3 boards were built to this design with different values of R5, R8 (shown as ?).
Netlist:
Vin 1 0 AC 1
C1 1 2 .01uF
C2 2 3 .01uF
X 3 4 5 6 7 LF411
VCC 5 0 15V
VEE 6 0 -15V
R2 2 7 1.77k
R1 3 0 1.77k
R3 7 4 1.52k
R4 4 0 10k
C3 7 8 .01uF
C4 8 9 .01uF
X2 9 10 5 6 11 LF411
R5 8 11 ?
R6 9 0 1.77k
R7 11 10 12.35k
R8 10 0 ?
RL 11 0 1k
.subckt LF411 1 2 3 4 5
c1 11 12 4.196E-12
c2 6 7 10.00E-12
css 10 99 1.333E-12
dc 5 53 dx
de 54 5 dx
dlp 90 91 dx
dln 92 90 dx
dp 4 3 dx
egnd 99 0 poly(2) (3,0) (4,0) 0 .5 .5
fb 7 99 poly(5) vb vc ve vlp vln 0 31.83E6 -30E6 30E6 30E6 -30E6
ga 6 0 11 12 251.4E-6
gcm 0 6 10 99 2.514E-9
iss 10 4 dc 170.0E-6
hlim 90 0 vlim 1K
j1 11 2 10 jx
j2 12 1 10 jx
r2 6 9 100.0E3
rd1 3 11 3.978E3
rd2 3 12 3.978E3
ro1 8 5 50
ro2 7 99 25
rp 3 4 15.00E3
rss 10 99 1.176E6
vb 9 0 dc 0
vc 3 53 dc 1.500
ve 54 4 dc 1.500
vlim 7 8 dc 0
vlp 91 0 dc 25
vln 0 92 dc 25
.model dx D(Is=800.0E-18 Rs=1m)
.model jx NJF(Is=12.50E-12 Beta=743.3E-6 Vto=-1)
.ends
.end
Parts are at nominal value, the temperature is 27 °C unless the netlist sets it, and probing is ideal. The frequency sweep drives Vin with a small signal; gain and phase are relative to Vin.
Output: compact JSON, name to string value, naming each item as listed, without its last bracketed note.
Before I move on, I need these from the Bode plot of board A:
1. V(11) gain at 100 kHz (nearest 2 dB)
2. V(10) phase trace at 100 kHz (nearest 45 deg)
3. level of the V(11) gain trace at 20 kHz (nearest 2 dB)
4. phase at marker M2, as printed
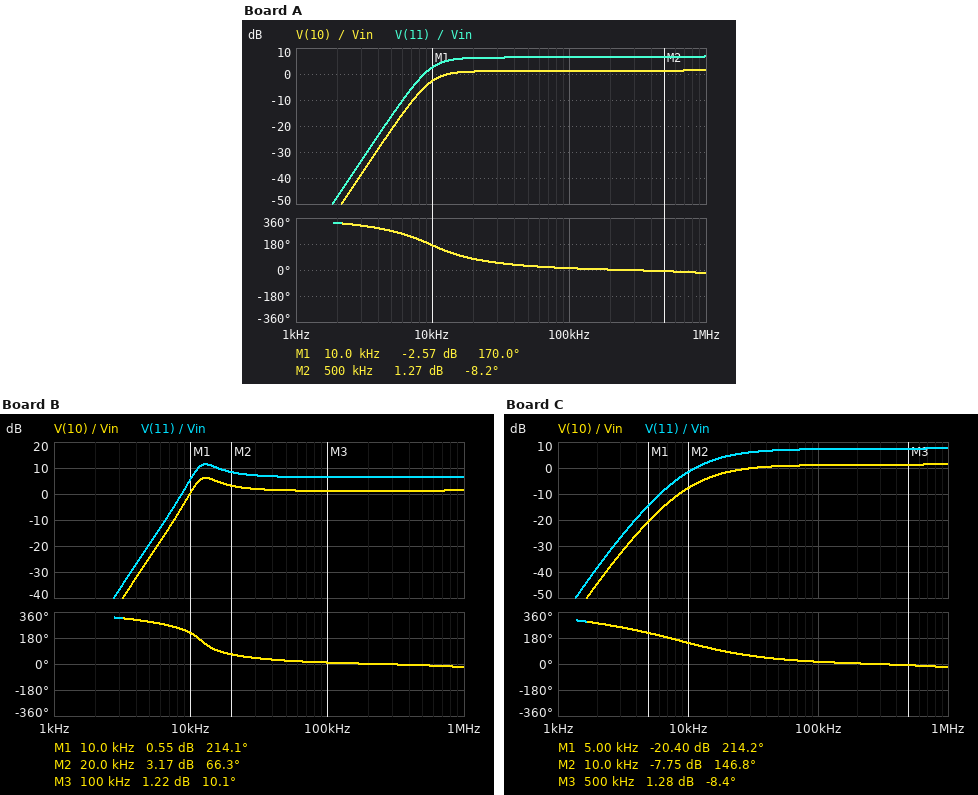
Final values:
{"V(11) gain at 100 kHz": "6 dB", "V(10) phase trace at 100 kHz": "0 deg", "level of the V(11) gain trace at 20 kHz": "6 dB", "phase at marker M2, as printed": "-8.2 deg"}
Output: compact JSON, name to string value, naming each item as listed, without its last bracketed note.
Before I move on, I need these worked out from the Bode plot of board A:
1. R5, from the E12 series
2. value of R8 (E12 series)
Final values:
{"R5, from the E12 series": "1.5 kΩ", "value of R8": "15 kΩ"}
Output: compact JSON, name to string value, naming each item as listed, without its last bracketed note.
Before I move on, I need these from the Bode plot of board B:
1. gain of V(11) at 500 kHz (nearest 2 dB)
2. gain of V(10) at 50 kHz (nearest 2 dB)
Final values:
{"gain of V(11) at 500 kHz": "6 dB", "gain of V(10) at 50 kHz": "2 dB"}
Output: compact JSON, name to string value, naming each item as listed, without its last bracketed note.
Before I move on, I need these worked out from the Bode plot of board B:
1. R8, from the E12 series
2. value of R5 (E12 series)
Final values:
{"R8, from the E12 series": "15 kΩ", "value of R5": "1 kΩ"}
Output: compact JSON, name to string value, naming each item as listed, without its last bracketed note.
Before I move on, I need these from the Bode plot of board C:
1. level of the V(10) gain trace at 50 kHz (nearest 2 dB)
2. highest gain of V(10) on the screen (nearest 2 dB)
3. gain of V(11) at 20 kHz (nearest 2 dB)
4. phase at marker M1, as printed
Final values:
{"level of the V(10) gain trace at 50 kHz": "0 dB", "highest gain of V(10) on the screen": "2 dB", "gain of V(11) at 20 kHz": "4 dB", "phase at marker M1, as printed": "214.2 deg"}
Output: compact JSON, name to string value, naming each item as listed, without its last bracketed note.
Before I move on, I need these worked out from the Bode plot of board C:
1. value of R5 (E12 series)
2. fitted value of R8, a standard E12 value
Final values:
{"value of R5": "5.6 kΩ", "fitted value of R8, a standard E12 value": "12 kΩ"}
